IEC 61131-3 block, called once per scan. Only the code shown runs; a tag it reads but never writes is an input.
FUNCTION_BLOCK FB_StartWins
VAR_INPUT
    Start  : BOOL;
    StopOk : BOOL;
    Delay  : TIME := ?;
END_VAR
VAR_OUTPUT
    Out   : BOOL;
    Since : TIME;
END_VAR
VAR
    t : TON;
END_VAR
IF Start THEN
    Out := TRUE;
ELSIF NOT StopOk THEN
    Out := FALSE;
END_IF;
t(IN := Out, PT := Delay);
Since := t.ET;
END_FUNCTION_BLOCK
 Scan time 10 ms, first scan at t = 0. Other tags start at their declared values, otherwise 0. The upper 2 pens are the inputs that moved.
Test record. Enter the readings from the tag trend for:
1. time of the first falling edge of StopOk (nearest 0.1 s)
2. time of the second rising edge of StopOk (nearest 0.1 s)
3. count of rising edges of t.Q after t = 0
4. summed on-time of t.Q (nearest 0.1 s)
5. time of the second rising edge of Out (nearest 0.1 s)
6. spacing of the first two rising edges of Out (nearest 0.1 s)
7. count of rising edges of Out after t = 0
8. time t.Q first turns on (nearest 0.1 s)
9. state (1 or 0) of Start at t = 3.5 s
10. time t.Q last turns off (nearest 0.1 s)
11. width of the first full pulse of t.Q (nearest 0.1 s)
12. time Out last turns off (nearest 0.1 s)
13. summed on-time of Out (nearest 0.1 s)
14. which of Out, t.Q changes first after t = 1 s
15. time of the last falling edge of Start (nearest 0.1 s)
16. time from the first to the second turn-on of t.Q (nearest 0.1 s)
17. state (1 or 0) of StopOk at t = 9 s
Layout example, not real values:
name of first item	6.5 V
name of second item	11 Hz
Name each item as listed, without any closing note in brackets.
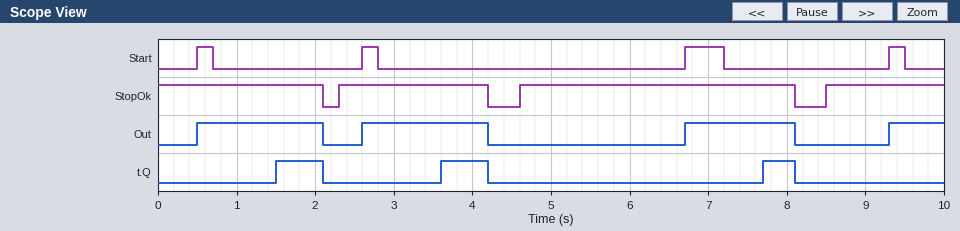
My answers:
time of the first falling edge of StopOk	2.1 s
time of the second rising edge of StopOk	4.6 s
count of rising edges of t.Q after t = 0	3
summed on-time of t.Q	1.6 s
time of the second rising edge of Out	2.6 s
spacing of the first two rising edges of Out	2.1 s
count of rising edges of Out after t = 0	4
time t.Q first turns on	1.5 s
state (1 or 0) of Start at t = 3.5 s	0
time t.Q last turns off	8.1 s
width of the first full pulse of t.Q	0.6 s
time Out last turns off	8.1 s
summed on-time of Out	5.3 s
which of Out, t.Q changes first after t = 1 s	t.Q
time of the last falling edge of Start	9.5 s
time from the first to the second turn-on of t.Q	2.1 s
state (1 or 0) of StopOk at t = 9 s	1
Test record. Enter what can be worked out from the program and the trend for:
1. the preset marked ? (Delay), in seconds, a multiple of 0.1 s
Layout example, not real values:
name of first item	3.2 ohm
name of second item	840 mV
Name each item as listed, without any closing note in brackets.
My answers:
the preset marked ? (Delay), in seconds, a multiple of 0.1 s	1.0 s
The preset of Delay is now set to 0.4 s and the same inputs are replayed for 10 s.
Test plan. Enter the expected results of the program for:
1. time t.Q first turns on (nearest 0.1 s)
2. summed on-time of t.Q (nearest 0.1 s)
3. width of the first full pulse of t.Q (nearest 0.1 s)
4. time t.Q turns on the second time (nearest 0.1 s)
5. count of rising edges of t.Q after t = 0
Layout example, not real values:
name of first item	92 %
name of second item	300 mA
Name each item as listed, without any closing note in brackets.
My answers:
time t.Q first turns on	0.9 s
summed on-time of t.Q	3.7 s
width of the first full pulse of t.Q	1.2 s
time t.Q turns on the second time	3.0 s
count of rising edges of t.Q after t = 0	4
